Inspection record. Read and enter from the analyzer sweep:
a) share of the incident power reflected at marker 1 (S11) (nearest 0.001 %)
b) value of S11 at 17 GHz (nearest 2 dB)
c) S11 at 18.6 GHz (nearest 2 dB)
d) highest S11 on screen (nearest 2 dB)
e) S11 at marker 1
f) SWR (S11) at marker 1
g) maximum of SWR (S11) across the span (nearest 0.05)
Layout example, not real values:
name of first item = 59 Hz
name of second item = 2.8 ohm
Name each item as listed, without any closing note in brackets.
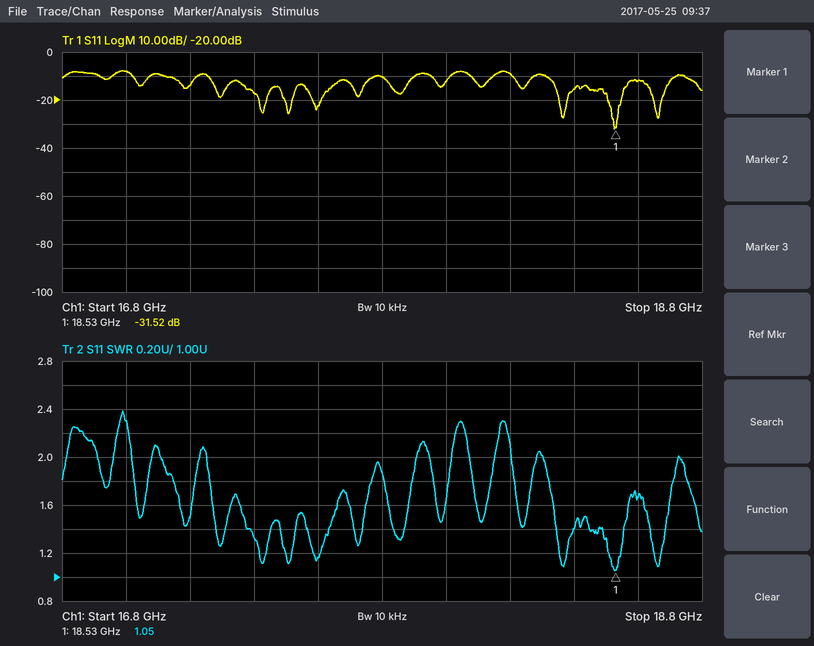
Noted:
share of the incident power reflected at marker 1 (S11) = 0.070 %
value of S11 at 17 GHz = -8 dB
S11 at 18.6 GHz = -12 dB
highest S11 on screen = -8 dB
S11 at marker 1 = -31.52 dB
SWR (S11) at marker 1 = 1.05
maximum of SWR (S11) across the span = 2.40
